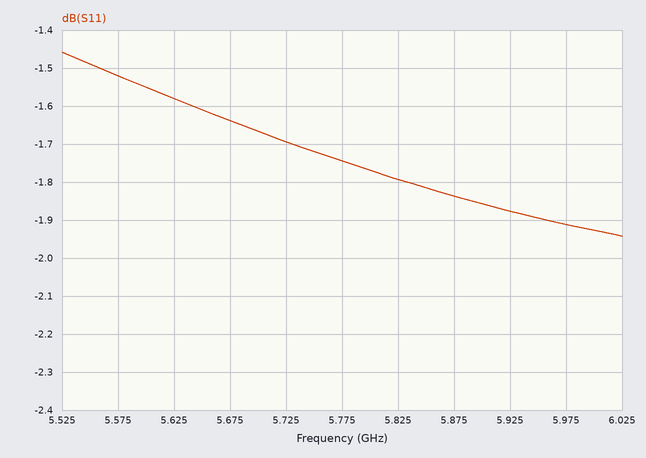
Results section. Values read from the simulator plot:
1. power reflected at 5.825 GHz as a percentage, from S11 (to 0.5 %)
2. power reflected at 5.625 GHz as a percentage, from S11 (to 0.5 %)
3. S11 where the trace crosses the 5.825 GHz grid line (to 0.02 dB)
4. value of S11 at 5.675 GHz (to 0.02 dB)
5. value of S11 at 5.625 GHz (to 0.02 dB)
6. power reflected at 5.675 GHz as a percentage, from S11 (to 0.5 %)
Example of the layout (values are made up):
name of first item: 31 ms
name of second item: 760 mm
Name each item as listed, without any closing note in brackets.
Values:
power reflected at 5.825 GHz as a percentage, from S11: 66.0 %
power reflected at 5.625 GHz as a percentage, from S11: 69.5 %
S11 where the trace crosses the 5.825 GHz grid line: -1.80 dB
value of S11 at 5.675 GHz: -1.64 dB
value of S11 at 5.625 GHz: -1.58 dB
power reflected at 5.675 GHz as a percentage, from S11: 68.5 %
